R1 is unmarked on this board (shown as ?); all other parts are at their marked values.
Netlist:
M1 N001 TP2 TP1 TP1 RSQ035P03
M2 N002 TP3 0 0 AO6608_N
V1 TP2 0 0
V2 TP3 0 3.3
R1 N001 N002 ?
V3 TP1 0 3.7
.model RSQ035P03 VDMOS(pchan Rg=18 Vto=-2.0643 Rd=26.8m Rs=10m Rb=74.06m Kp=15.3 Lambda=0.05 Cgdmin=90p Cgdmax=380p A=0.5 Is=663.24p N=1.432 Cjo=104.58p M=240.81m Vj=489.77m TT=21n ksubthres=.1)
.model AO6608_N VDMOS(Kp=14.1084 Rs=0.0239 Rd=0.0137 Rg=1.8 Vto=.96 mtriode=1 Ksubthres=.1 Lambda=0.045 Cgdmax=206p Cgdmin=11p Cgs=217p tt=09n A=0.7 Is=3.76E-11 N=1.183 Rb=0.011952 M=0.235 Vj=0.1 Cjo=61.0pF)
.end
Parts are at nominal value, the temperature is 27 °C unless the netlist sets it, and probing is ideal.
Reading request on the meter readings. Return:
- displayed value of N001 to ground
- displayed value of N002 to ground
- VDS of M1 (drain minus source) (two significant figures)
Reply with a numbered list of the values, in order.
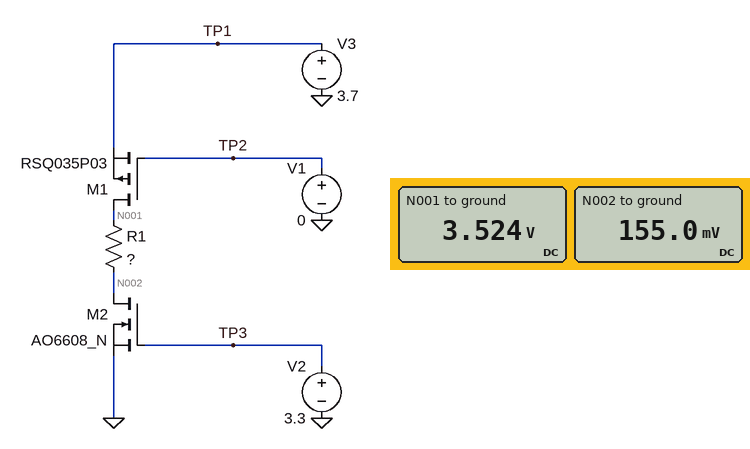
1. 3.524 V
2. 155.0 mV
3. -180 mV
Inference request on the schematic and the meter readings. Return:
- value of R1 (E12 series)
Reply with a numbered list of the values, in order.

1. 1.5 Ω
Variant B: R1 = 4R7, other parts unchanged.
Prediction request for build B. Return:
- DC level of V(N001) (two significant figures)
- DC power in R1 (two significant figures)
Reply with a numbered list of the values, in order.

1. 3.6 V
2. 2.7 W
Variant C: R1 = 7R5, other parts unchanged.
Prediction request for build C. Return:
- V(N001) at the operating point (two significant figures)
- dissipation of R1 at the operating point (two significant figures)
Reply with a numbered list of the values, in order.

1. 3.7 V
2. 1.8 W
